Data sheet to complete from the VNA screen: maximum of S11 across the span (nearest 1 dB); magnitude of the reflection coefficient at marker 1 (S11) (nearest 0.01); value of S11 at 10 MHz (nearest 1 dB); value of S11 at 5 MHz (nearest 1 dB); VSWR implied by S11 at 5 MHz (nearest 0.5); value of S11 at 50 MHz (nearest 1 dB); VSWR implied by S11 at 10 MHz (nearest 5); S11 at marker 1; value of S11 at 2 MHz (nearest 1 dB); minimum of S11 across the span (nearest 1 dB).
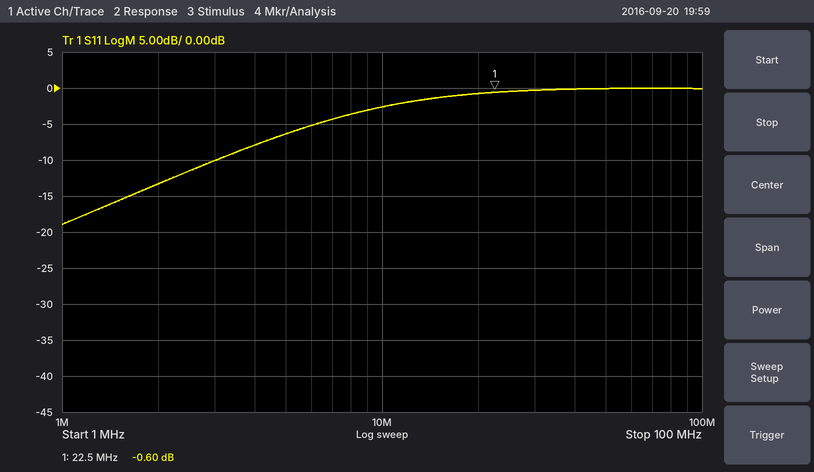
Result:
0 dB
0.93
-3 dB
-6 dB
3.0
0 dB
5
-0.60 dB
-13 dB
-19 dB
